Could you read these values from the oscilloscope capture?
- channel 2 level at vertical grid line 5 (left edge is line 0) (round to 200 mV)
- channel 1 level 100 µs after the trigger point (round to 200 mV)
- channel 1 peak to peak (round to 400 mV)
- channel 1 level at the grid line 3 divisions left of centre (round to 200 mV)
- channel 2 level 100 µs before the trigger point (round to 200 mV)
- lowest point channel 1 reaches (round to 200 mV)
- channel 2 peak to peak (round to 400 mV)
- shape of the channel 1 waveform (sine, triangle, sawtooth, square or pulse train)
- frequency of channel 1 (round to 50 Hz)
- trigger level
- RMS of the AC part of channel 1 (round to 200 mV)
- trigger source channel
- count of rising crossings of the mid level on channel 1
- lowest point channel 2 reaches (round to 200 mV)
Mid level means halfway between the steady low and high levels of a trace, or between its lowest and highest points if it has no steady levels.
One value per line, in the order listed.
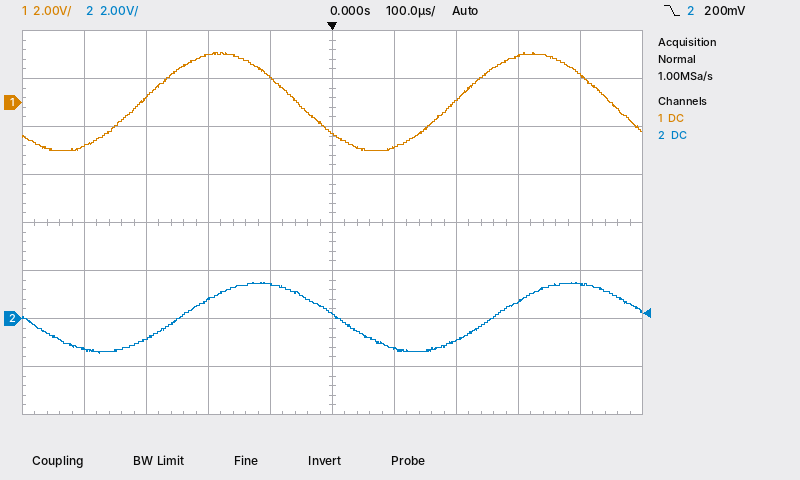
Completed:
200 mV
-1.8 V
4.0 V
200 mV
1.4 V
-2.0 V
2.8 V
sine
2.00 kHz
200 mV
1.4 V
channel 2
2
-1.4 V
